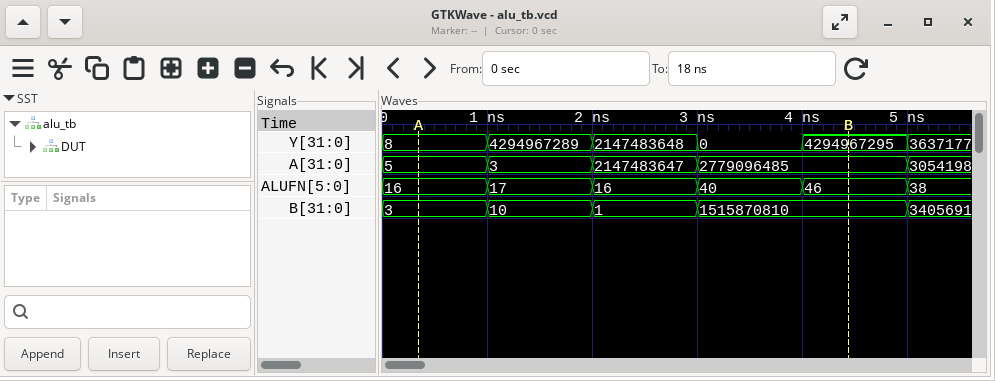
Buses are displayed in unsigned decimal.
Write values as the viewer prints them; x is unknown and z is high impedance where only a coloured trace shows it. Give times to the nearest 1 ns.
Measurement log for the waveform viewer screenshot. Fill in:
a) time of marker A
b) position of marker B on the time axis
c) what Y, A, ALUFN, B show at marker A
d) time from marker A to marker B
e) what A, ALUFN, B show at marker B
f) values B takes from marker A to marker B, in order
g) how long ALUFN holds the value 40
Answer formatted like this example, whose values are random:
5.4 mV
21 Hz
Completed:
0 ns
4 ns
Y=8, A=5, ALUFN=16, B=3
4 ns
A=2779096485, ALUFN=46, B=1515870810
3, 10, 1, 1515870810
1 ns
